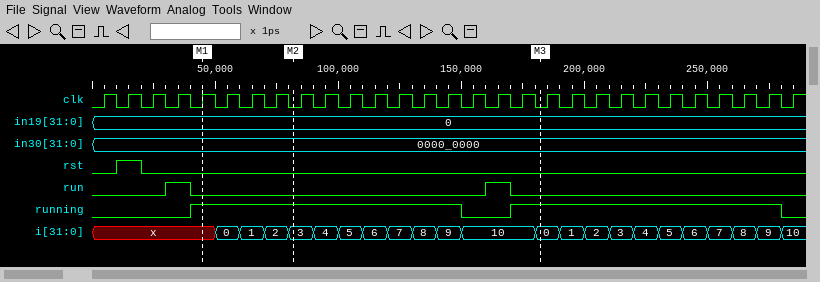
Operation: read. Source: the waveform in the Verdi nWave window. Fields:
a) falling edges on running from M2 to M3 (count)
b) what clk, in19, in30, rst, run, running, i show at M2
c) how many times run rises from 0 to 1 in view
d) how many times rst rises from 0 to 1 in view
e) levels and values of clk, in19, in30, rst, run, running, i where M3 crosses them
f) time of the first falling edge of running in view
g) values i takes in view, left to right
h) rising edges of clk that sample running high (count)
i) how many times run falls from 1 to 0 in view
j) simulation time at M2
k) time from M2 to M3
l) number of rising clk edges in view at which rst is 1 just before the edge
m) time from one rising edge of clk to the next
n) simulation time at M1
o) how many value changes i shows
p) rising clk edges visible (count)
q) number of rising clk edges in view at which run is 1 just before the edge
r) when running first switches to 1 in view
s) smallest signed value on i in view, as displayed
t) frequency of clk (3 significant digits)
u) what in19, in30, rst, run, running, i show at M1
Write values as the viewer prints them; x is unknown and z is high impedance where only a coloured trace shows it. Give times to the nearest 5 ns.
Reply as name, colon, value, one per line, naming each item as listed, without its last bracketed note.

falling edges on running from M2 to M3: 1
what clk, in19, in30, rst, run, running, i show at M2: clk=0, in19=0, in30=0000_0000, rst=0, run=0, running=1, i=3
how many times run rises from 0 to 1 in view: 2
how many times rst rises from 0 to 1 in view: 1
levels and values of clk, in19, in30, rst, run, running, i where M3 crosses them: clk=0, in19=0, in30=0000_0000, rst=0, run=0, running=1, i=0
time of the first falling edge of running in view: 150 ns
values i takes in view, left to right: x, 0, 1, 2, 3, 4, 5, 6, 7, 8, 9, 10, 0, 1, 2, 3, 4, 5, 6, 7, 8, 9, 10
rising edges of clk that sample running high: 22
how many times run falls from 1 to 0 in view: 2
simulation time at M2: 80 ns
time from M2 to M3: 100 ns
number of rising clk edges in view at which rst is 1 just before the edge: 1
time from one rising edge of clk to the next: 10 ns
simulation time at M1: 45 ns
how many value changes i shows: 22
rising clk edges visible: 29
number of rising clk edges in view at which run is 1 just before the edge: 2
when running first switches to 1 in view: 40 ns
smallest signed value on i in view, as displayed: 0
frequency of clk: 100 MHz
what in19, in30, rst, run, running, i show at M1: in19=0, in30=0000_0000, rst=0, run=0, running=1, i=x
